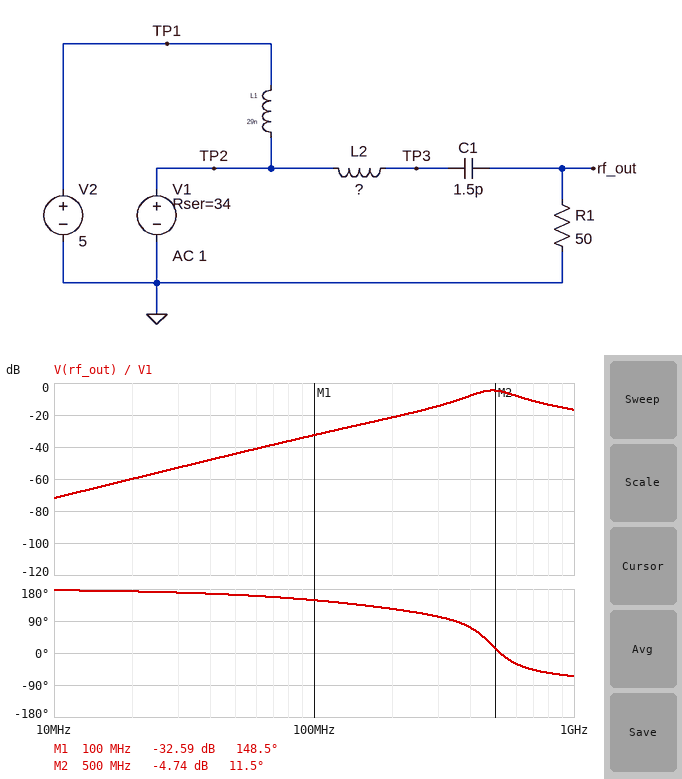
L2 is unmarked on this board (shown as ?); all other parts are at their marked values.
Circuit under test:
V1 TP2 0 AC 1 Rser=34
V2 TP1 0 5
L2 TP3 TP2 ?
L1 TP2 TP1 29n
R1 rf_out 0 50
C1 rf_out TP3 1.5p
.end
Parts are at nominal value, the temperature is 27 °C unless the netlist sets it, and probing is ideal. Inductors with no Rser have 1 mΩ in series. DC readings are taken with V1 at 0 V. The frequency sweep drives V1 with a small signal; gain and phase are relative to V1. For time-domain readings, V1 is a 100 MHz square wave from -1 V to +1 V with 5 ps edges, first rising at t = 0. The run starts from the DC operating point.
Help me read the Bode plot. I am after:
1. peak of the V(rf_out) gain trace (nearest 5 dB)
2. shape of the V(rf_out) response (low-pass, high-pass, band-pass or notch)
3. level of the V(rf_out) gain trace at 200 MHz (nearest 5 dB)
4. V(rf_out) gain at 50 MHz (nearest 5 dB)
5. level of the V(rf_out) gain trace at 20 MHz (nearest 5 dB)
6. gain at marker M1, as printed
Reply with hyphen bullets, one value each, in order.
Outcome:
- -5 dB
- band-pass
- -20 dB
- -45 dB
- -60 dB
- -32.59 dB
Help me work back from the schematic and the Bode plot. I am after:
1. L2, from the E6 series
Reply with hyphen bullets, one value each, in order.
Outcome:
- 68 nH
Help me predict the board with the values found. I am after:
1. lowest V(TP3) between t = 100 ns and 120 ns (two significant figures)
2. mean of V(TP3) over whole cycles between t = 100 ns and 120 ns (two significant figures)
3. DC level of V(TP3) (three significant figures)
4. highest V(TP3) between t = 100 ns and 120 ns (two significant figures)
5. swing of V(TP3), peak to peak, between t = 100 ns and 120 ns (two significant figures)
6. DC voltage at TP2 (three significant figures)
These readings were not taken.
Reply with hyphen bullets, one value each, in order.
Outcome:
- 3.0 V
- 5.0 V
- 5.00 V
- 7.0 V
- 4.0 V
- 5.00 V
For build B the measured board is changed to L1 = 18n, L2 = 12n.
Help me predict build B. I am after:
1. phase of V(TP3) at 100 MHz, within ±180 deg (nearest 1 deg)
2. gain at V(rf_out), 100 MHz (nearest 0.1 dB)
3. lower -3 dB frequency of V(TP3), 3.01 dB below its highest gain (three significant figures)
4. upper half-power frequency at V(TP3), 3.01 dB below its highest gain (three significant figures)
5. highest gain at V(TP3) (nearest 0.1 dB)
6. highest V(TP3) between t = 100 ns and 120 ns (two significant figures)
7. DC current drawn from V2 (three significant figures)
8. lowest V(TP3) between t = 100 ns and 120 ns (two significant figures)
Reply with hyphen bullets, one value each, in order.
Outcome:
- 71 deg
- -36.4 dB
- 414 MHz
- 1.43 GHz
- 2.6 dB
- 6.8 V
- 147 mA
- 3.2 V
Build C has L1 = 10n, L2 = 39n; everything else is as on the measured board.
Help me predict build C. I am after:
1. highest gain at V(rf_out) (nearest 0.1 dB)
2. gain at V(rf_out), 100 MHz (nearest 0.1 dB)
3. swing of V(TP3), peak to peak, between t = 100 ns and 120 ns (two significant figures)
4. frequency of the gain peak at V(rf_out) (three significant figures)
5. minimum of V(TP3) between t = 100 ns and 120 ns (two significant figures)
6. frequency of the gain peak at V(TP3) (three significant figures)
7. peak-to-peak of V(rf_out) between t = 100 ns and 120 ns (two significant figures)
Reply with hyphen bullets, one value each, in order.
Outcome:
- -5.3 dB
- -41.1 dB
- 2.6 V
- 630 MHz
- 3.7 V
- 604 MHz
- 520 mV
